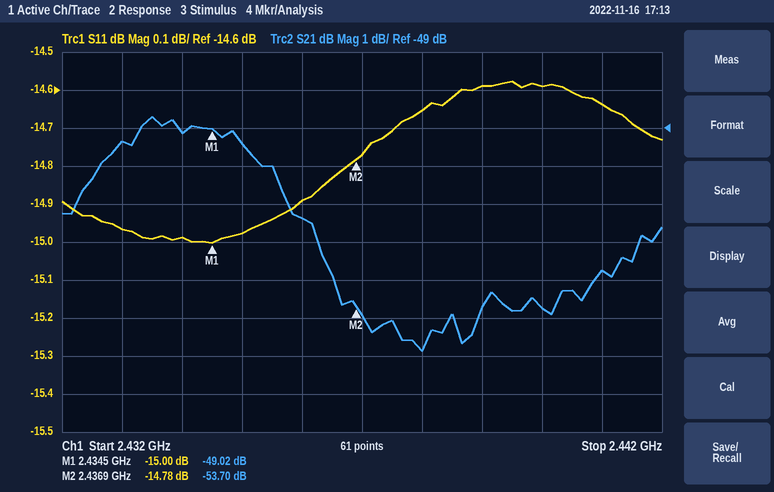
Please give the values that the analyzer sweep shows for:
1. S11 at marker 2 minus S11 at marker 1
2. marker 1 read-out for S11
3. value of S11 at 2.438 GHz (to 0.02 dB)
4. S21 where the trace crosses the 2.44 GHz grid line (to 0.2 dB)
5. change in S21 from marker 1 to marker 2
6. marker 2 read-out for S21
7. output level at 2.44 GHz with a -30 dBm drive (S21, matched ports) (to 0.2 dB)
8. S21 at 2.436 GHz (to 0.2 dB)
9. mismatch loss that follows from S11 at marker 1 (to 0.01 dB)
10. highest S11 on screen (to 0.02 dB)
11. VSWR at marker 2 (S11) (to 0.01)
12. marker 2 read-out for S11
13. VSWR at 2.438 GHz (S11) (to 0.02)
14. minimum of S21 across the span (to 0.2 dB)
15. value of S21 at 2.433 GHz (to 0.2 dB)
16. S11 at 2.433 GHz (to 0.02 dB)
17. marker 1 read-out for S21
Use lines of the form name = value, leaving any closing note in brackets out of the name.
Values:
S11 at marker 2 minus S11 at marker 1 = 0.22 dB
marker 1 read-out for S11 = -15.00 dB
value of S11 at 2.438 GHz = -14.66 dB
S21 where the trace crosses the 2.44 GHz grid line = -53.8 dB
change in S21 from marker 1 to marker 2 = -4.68 dB
marker 2 read-out for S21 = -53.70 dB
output level at 2.44 GHz with a -30 dBm drive (S21, matched ports) = -83.8 dBm
S21 at 2.436 GHz = -51.4 dB
mismatch loss that follows from S11 at marker 1 = 0.14 dB
highest S11 on screen = -14.58 dB
VSWR at marker 2 (S11) = 1.45
marker 2 read-out for S11 = -14.78 dB
VSWR at 2.438 GHz (S11) = 1.46
minimum of S21 across the span = -54.8 dB
value of S21 at 2.433 GHz = -49.4 dB
S11 at 2.433 GHz = -14.96 dB
marker 1 read-out for S21 = -49.02 dB
